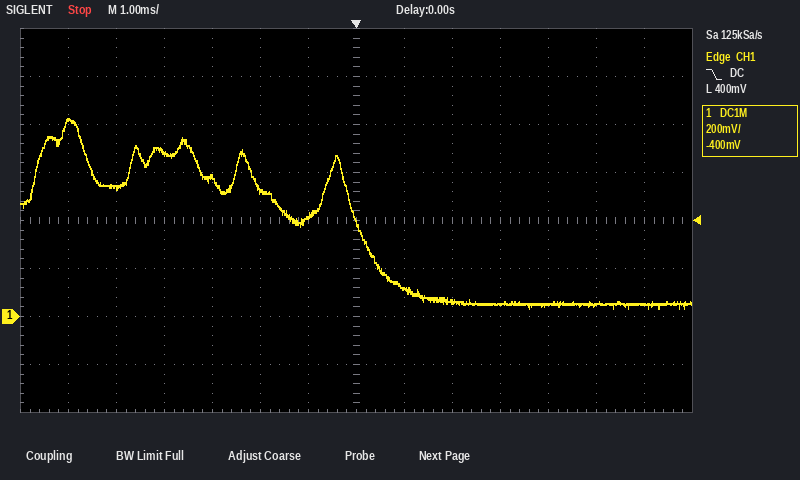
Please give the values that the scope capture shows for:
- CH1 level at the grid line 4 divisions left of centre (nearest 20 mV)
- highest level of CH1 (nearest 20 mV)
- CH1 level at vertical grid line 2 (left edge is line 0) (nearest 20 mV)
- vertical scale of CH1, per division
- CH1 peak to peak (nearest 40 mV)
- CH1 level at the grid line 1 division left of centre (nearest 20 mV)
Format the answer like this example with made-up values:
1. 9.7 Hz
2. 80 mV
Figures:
1. 680 mV
2. 820 mV
3. 540 mV
4. 200 mV
5. 800 mV
6. 420 mV
